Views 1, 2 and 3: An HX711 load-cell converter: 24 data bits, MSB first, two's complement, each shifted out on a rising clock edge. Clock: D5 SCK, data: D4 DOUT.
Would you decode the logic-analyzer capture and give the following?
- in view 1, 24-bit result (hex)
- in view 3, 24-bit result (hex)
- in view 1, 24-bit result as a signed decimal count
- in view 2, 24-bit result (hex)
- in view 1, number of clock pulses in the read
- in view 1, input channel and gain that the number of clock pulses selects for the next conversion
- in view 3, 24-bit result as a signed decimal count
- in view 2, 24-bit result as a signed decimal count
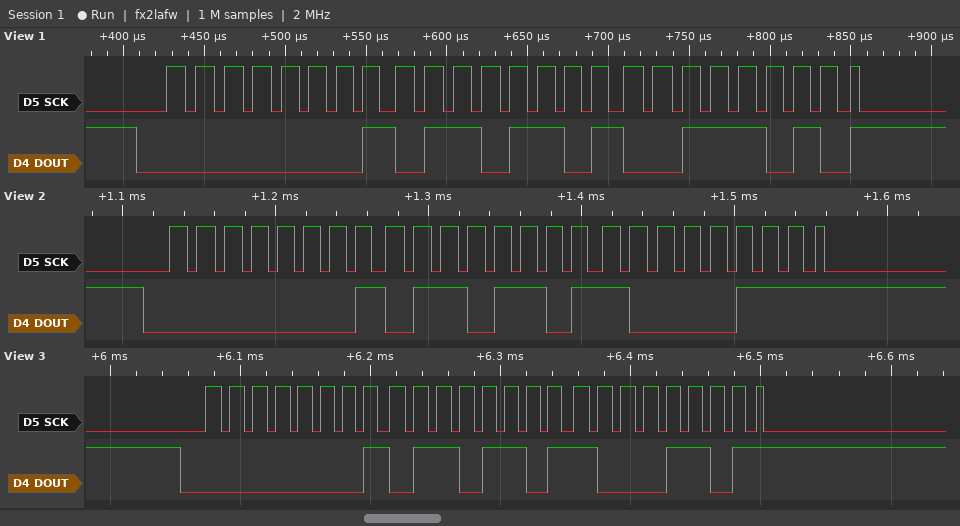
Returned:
0x016D3A
0x016D8D
93498
0x016D87
25
channel A, gain 128
93581
93575
